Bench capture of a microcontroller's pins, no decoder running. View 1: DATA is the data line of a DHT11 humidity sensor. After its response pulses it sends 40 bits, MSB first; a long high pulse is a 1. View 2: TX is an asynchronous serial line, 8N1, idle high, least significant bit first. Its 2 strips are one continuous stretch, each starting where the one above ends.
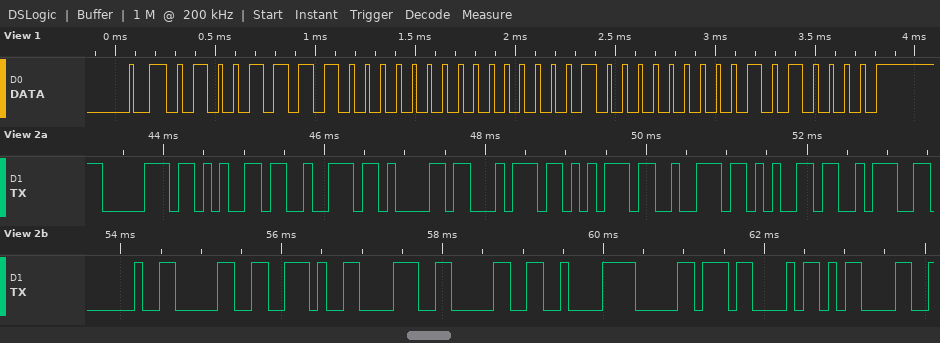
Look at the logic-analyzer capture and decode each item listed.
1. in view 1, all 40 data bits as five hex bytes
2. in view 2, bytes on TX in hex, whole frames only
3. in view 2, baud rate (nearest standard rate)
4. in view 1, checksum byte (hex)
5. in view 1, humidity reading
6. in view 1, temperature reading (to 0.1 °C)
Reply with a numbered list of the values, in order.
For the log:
1. 4F 00 01 00 50
2. 70 65 72 61 74 75 72 65 3A 20 30 2E 38 30 C2 B0 43 0D
3. 9600 baud
4. 0x50
5. 79 %
6. 1.0 °C
